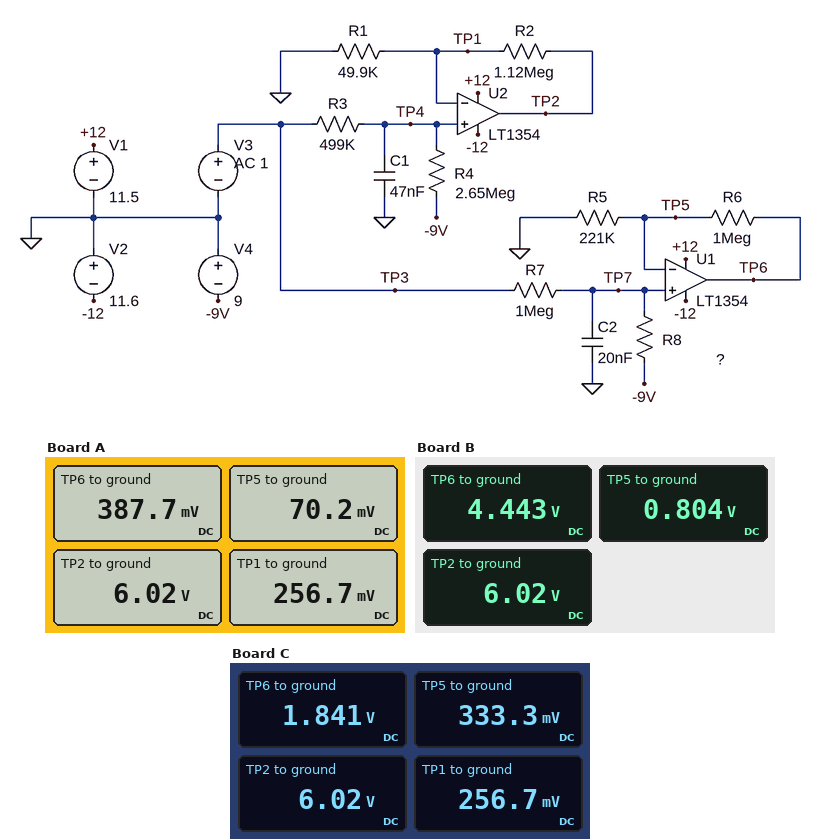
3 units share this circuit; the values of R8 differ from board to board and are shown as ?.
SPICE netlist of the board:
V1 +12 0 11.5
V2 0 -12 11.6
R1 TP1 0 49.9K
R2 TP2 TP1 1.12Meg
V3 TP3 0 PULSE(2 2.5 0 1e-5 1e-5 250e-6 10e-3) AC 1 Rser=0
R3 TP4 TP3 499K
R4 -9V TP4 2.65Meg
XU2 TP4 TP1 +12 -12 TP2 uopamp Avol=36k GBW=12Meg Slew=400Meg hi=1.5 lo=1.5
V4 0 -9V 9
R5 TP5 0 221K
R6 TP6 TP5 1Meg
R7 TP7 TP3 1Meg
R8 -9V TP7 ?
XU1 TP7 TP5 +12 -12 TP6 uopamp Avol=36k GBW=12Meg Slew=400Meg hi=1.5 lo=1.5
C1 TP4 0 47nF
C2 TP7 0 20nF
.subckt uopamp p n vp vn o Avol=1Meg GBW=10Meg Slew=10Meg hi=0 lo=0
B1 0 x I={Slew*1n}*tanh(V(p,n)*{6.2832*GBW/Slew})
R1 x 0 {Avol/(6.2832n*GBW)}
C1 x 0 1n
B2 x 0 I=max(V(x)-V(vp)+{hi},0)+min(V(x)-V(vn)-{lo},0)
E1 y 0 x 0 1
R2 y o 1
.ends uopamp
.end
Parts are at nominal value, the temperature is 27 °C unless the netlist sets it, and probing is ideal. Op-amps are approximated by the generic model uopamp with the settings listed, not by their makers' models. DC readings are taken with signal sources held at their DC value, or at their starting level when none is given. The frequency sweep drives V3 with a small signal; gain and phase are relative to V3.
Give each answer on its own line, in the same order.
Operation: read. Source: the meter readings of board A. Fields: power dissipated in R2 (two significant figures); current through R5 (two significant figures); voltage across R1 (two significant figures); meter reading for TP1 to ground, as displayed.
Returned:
30 µW
320 nA
260 mV
256.7 mV
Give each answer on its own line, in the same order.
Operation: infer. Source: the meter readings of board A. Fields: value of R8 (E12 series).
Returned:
4.7 MΩ
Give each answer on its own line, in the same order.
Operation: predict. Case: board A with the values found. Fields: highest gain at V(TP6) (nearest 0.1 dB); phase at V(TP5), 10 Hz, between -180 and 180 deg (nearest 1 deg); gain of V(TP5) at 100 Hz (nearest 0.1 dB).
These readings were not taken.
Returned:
13.2 dB
-46 deg
-22.0 dB
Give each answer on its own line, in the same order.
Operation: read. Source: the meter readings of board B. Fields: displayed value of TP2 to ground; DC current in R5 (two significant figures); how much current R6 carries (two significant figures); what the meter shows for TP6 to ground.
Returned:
6.02 V
3.6 µA
3.6 µA
4.443 V
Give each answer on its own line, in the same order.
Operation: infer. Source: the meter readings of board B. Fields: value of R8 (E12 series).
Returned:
8.2 MΩ
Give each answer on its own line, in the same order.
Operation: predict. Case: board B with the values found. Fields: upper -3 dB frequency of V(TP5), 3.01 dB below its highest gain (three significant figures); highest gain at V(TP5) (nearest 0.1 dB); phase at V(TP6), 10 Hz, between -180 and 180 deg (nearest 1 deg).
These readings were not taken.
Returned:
8.93 Hz
-1.0 dB
-48 deg
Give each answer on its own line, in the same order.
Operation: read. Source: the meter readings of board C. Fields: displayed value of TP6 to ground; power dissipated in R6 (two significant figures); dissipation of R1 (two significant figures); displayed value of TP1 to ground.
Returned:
1.841 V
2.3 µW
1.3 µW
256.7 mV
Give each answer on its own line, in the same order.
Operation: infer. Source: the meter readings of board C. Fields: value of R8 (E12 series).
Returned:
5.6 MΩ
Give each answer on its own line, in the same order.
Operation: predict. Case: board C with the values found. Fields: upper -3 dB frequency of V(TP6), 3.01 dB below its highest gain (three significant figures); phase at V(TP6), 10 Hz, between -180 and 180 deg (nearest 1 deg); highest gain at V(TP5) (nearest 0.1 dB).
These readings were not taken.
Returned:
9.38 Hz
-47 deg
-1.4 dB
